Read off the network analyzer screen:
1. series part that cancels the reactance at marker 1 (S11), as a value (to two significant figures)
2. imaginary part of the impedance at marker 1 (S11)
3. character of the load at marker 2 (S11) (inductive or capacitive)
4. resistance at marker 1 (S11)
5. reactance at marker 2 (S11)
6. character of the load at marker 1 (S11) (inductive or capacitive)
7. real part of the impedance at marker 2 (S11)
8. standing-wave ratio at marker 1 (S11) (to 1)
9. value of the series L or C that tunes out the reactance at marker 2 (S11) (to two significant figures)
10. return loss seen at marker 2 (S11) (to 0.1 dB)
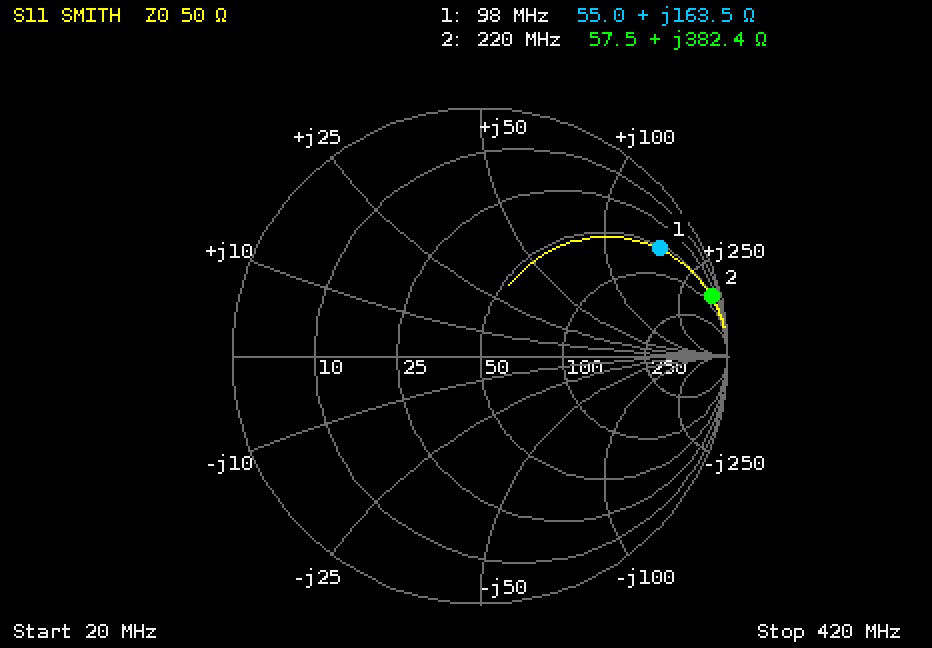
9.9 pF
+163.5 Ω
inductive
55.0 Ω
+382.4 Ω
inductive
57.5 Ω
12
1.9 pF
0.3 dB
